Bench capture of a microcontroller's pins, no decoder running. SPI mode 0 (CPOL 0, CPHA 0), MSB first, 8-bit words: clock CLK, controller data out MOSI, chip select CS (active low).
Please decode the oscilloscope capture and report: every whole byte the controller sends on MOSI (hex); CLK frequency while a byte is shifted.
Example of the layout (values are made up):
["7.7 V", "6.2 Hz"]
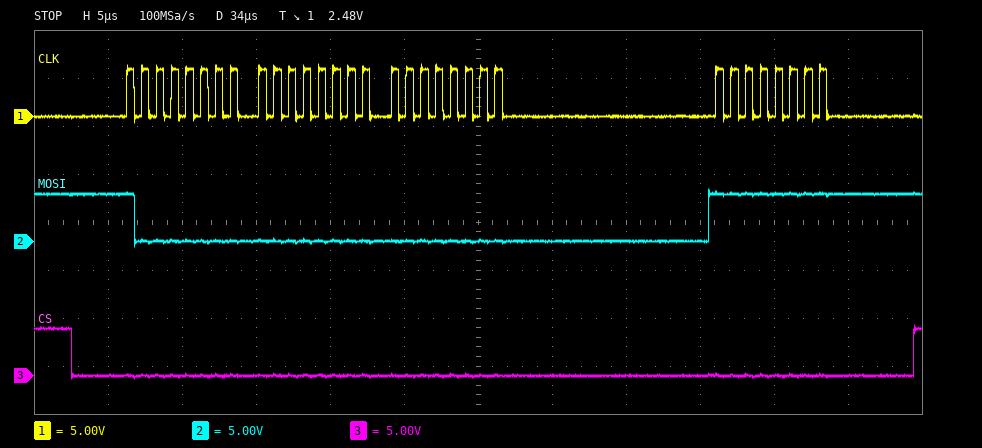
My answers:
["80 00 00 FF", "1 MHz"]
